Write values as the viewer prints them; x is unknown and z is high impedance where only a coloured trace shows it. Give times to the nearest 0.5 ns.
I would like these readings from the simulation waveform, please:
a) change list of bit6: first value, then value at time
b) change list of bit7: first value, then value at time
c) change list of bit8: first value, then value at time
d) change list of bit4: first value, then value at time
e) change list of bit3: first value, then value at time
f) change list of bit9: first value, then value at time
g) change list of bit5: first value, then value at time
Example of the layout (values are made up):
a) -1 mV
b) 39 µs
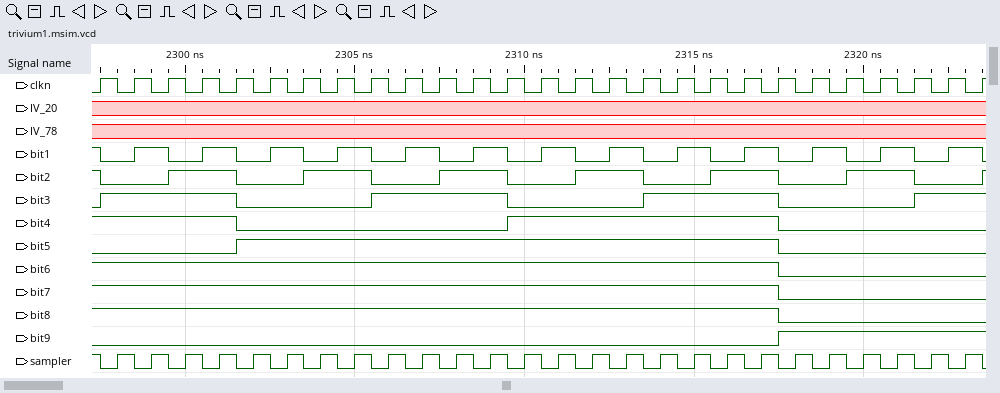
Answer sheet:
a) 1, 0 at 2317.5 ns
b) 1, 0 at 2317.5 ns
c) 1, 0 at 2317.5 ns
d) 1, 0 at 2301.5 ns, 1 at 2309.5 ns, 0 at 2317.5 ns
e) 0, 1 at 2297.5 ns, 0 at 2301.5 ns, 1 at 2305.5 ns, 0 at 2309.5 ns, 1 at 2313.5 ns, 0 at 2317.5 ns, 1 at 2321.5 ns
f) 0, 1 at 2317.5 ns
g) 0, 1 at 2301.5 ns, 0 at 2317.5 ns
